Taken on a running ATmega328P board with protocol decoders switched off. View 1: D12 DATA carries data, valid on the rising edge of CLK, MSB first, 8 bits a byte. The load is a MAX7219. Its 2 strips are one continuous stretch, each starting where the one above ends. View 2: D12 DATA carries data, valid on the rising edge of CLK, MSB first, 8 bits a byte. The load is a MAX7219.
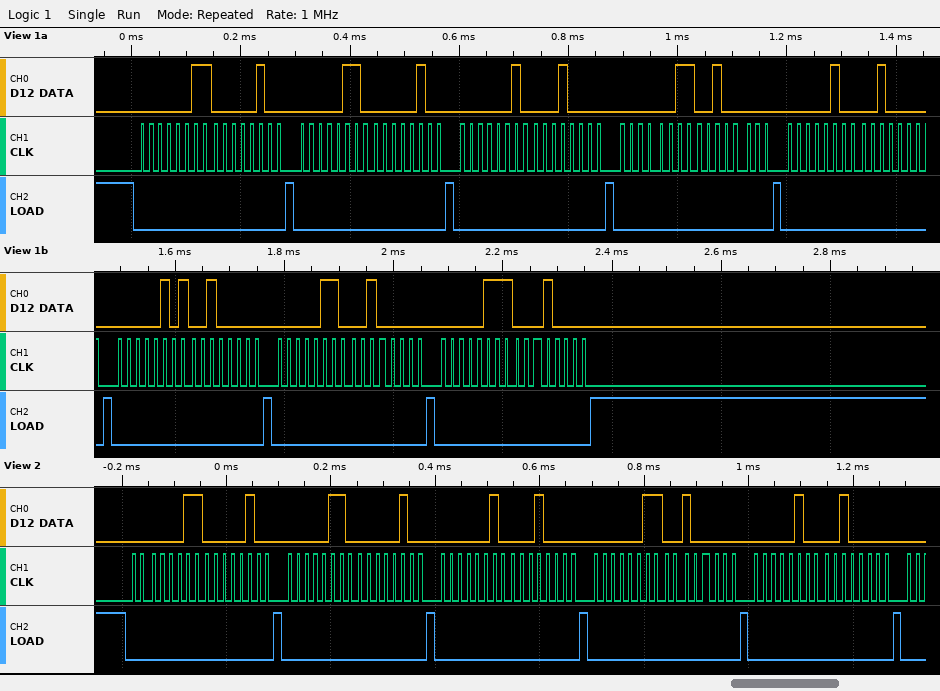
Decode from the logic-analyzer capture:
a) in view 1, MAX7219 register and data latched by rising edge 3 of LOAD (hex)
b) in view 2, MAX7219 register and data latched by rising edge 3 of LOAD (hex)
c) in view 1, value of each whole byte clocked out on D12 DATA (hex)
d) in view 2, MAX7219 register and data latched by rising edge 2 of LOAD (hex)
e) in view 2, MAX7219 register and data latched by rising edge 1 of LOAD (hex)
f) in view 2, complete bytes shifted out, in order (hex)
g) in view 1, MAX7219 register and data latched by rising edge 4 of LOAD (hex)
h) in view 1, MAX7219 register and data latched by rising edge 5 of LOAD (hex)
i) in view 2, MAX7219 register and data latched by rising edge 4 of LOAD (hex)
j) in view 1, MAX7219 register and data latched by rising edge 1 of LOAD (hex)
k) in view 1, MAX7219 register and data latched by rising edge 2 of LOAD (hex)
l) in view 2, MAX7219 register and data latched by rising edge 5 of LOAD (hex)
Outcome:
register 0x2, data 0x10
register 0x2, data 0x10
03 04 06 04 02 10 03 20 04 20 05 20 06 20 07 10
register 0x6, data 0x04
register 0x3, data 0x04
03 04 06 04 02 10 03 20 04 20
register 0x3, data 0x20
register 0x4, data 0x20
register 0x3, data 0x20
register 0x3, data 0x04
register 0x6, data 0x04
register 0x4, data 0x20
